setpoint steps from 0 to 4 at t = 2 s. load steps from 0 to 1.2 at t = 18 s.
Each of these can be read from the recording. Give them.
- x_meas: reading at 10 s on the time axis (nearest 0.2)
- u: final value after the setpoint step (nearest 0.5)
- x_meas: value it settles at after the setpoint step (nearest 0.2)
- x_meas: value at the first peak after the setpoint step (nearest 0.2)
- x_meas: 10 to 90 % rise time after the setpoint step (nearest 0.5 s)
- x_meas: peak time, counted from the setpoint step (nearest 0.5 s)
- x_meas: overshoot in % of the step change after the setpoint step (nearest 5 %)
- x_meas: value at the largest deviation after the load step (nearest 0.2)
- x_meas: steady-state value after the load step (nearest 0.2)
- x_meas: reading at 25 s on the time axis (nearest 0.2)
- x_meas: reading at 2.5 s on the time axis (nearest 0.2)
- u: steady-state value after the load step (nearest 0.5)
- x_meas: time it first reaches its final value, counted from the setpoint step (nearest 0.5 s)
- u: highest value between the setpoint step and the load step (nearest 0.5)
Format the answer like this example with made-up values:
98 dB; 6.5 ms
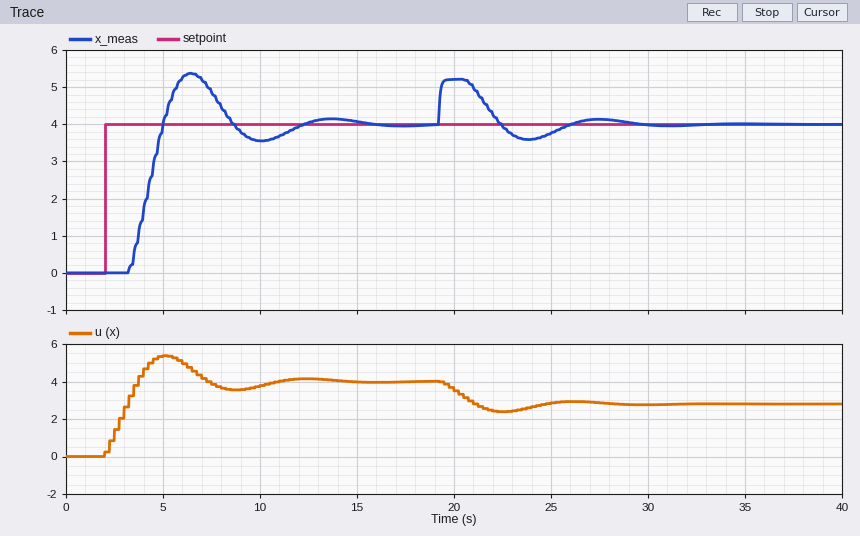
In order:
3.6; 4.0; 4.0; 5.4; 1.5 s; 4.5 s; 35 %; 5.2; 4.0; 3.8; 0.0; 3.0; 3.0 s; 5.5
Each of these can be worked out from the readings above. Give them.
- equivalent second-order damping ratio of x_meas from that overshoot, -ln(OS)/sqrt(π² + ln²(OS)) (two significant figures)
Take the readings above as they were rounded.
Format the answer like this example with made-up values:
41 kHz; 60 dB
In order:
0.32
